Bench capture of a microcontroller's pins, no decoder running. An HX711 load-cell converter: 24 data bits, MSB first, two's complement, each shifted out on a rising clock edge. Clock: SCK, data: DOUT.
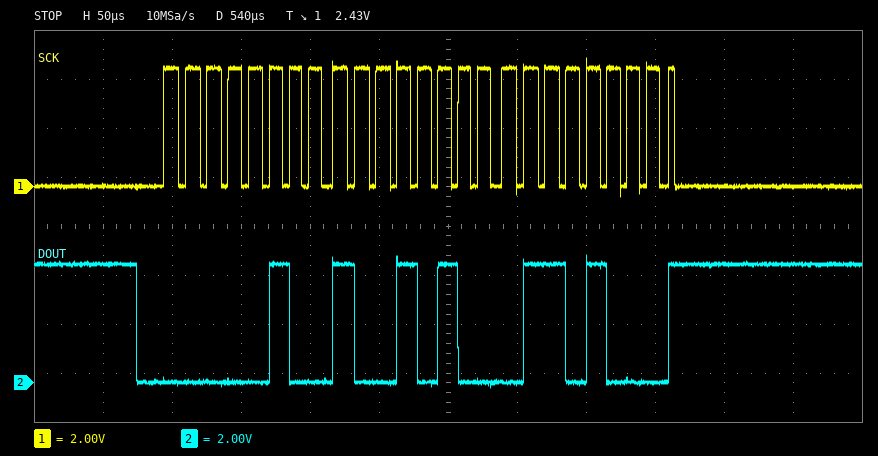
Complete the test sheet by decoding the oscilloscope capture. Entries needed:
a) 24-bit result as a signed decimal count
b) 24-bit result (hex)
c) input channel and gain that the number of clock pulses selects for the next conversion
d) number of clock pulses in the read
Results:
300136
0x049468
channel A, gain 128
25
